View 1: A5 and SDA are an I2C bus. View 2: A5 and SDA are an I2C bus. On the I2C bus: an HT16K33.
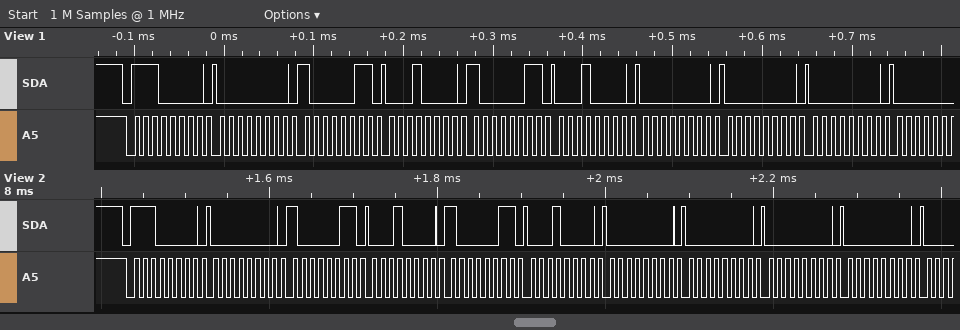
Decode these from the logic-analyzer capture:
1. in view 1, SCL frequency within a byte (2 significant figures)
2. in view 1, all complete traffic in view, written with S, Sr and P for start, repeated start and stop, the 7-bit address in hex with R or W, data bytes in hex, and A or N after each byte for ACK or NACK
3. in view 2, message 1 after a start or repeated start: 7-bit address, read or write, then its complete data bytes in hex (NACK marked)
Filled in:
100 kHz
S 70W A 00 A 83 A 10 A 83 A 10 A 00 A 00 A 00 A
0x70 write: 00 83 10 83 10 00 00 00 00
